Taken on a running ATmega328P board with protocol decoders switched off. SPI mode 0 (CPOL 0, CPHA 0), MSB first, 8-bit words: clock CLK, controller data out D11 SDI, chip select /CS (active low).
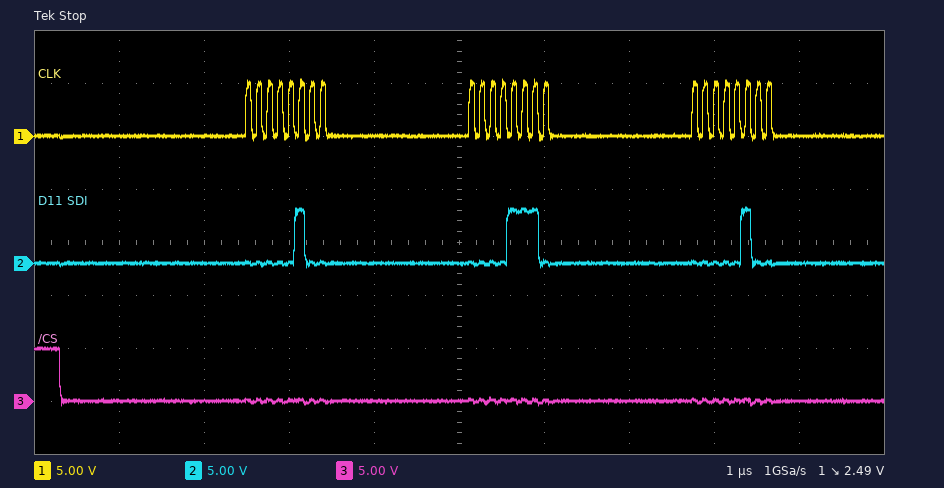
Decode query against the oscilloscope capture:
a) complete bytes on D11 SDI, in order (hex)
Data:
04 0E 04
